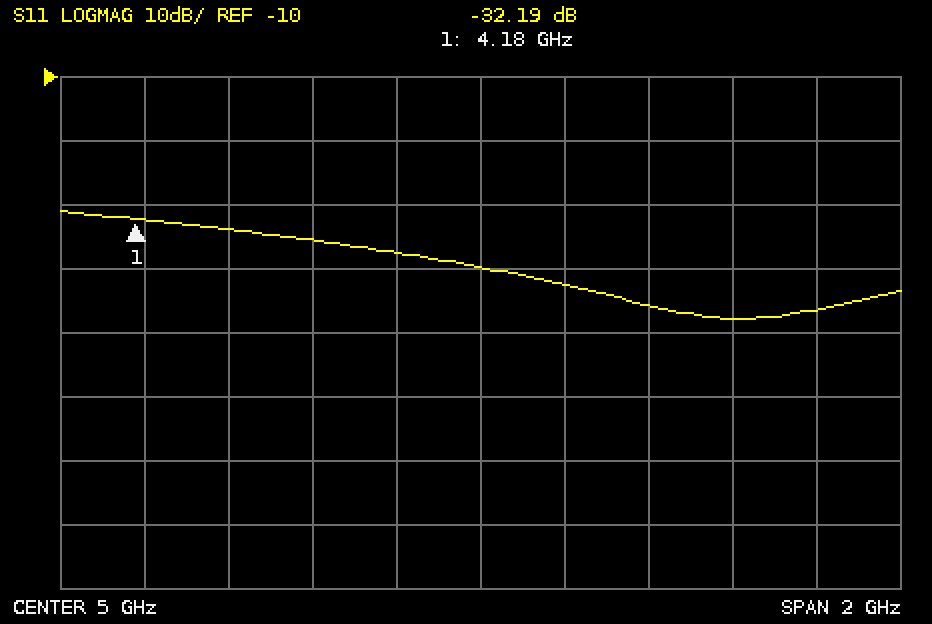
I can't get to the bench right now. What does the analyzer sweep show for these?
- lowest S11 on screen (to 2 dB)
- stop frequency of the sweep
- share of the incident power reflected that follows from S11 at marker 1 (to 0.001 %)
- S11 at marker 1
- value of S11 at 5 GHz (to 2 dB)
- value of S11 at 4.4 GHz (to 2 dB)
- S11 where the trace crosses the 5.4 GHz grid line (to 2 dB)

-48 dB
6 GHz
0.060 %
-32.19 dB
-40 dB
-34 dB
-46 dB
